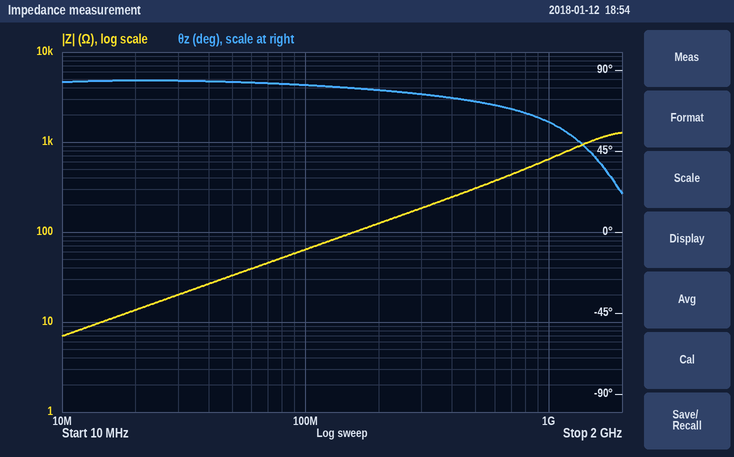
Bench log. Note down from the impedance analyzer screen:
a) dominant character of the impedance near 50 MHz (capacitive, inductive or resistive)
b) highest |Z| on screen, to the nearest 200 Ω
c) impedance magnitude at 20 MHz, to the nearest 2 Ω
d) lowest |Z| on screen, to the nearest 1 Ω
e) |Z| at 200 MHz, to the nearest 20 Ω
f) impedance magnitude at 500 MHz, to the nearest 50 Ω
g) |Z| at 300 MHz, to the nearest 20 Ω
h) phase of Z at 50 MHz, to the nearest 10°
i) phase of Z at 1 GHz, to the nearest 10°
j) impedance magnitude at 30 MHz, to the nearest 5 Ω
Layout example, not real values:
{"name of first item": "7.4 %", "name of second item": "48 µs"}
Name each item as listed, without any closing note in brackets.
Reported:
{"dominant character of the impedance near 50 MHz": "inductive", "highest |Z| on screen, to the nearest 200 Ω": "1.2 kΩ", "impedance magnitude at 20 MHz, to the nearest 2 Ω": "14 Ω", "lowest |Z| on screen, to the nearest 1 Ω": "7 Ω", "|Z| at 200 MHz, to the nearest 20 Ω": "120 Ω", "impedance magnitude at 500 MHz, to the nearest 50 Ω": "300 Ω", "|Z| at 300 MHz, to the nearest 20 Ω": "180 Ω", "phase of Z at 50 MHz, to the nearest 10°": "80°", "phase of Z at 1 GHz, to the nearest 10°": "60°", "impedance magnitude at 30 MHz, to the nearest 5 Ω": "20 Ω"}
